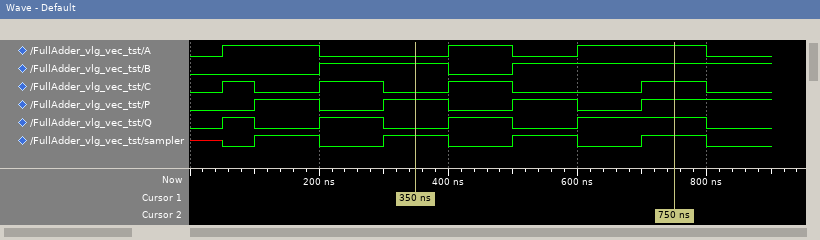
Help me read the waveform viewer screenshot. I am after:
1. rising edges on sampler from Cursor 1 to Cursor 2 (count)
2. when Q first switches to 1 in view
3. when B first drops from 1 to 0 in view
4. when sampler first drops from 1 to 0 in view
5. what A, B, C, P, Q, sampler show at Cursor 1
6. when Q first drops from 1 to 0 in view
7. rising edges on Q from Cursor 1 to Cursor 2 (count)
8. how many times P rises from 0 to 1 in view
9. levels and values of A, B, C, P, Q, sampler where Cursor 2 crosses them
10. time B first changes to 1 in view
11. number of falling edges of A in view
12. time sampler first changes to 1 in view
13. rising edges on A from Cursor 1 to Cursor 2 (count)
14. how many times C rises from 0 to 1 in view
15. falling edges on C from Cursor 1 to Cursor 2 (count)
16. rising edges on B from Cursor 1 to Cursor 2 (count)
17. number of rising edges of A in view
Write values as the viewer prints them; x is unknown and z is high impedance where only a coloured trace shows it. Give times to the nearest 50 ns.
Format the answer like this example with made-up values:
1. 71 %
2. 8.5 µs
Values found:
1. 2
2. 50 ns
3. 400 ns
4. 200 ns
5. A=0, B=1, C=0, P=1, Q=0, sampler=1
6. 100 ns
7. 2
8. 4
9. A=1, B=1, C=1, P=1, Q=1, sampler=1
10. 200 ns
11. 3
12. 100 ns
13. 2
14. 4
15. 1
16. 1
17. 3
